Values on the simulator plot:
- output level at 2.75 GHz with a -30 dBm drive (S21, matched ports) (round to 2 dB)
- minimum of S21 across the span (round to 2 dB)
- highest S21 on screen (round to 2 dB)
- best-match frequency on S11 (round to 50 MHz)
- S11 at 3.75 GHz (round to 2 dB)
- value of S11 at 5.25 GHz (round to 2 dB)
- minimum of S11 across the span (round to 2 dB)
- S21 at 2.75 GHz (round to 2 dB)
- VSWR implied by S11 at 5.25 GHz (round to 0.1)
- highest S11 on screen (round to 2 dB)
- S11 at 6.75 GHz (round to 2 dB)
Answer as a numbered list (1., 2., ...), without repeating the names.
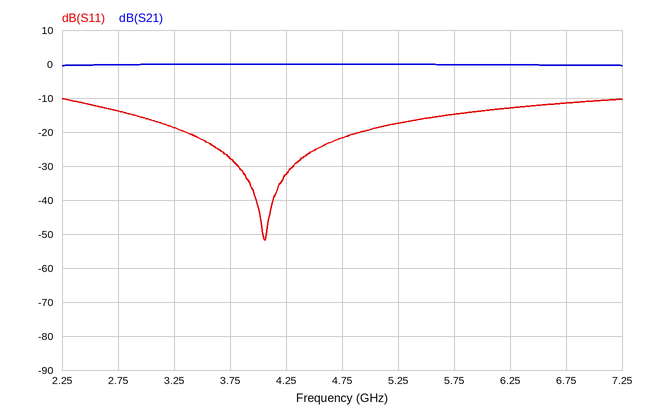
1. -30 dBm
2. 0 dB
3. 0 dB
4. 4.05 GHz
5. -28 dB
6. -18 dB
7. -52 dB
8. 0 dB
9. 1.3
10. -10 dB
11. -12 dB
